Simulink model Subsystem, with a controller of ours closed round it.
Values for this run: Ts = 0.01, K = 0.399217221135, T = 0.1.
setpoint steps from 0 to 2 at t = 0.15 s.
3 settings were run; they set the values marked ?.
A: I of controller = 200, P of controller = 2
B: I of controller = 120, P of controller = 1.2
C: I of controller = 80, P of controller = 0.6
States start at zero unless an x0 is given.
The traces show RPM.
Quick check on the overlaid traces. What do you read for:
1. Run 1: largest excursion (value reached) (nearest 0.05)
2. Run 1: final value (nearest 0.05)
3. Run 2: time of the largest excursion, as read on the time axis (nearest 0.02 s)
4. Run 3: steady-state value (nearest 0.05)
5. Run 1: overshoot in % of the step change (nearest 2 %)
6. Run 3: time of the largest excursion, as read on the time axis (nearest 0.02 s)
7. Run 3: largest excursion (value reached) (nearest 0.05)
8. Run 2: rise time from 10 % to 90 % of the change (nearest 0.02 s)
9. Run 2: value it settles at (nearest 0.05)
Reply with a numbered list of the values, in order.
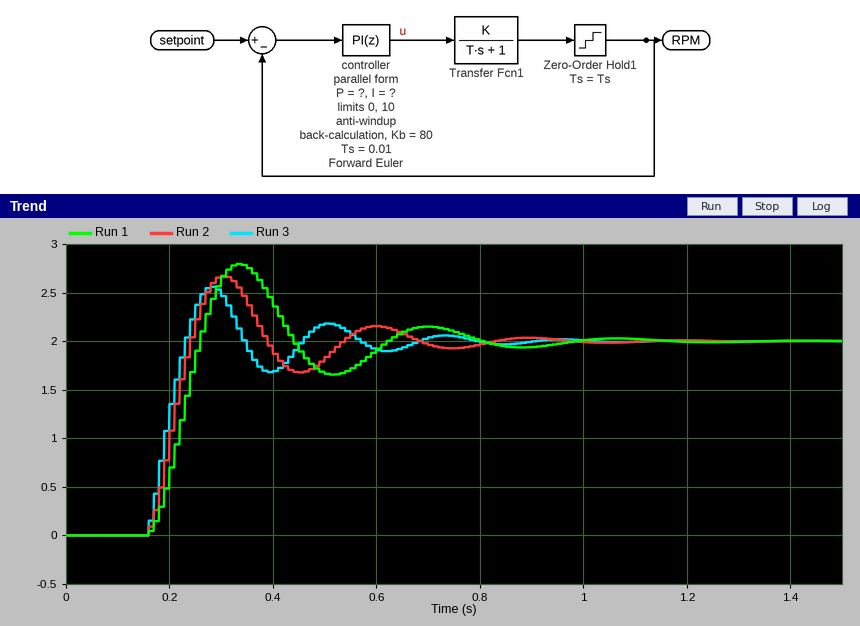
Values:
1. 2.80
2. 2.00
3. 0.30 s
4. 2.00
5. 40 %
6. 0.28 s
7. 2.55
8. 0.06 s
9. 2.00
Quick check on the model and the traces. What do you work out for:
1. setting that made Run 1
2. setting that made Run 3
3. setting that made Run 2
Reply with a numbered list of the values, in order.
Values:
1. C
2. A
3. B
